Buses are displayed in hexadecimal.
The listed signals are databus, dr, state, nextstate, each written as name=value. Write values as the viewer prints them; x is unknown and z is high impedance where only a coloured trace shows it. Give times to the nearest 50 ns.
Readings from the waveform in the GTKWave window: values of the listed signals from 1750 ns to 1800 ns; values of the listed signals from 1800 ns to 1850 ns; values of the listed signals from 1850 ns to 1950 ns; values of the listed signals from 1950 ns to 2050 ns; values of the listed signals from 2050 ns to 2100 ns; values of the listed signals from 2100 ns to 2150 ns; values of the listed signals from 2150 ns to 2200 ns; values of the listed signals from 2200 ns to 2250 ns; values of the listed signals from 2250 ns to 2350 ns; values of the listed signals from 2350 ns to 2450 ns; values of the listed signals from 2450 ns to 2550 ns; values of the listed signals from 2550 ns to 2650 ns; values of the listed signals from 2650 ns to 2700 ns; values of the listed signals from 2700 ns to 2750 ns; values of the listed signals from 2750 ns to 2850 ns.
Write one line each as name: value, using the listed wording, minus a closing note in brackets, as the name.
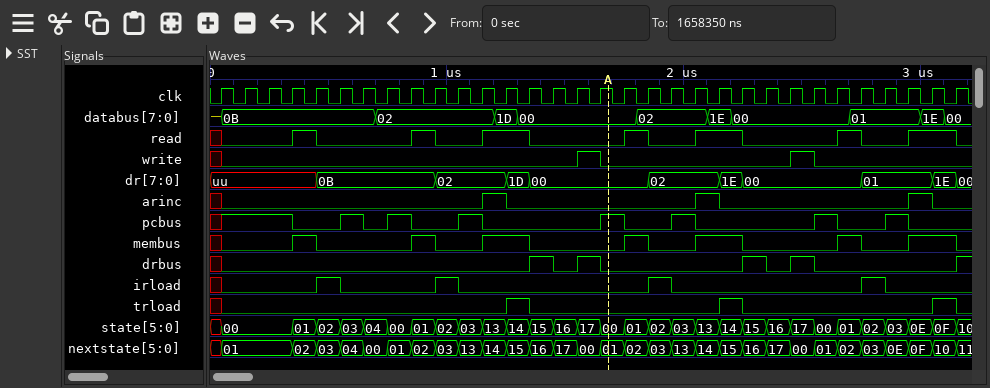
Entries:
values of the listed signals from 1750 ns to 1800 ns: databus=00, dr=00, state=01, nextstate=02
values of the listed signals from 1800 ns to 1850 ns: databus=02, dr=00, state=01, nextstate=02
values of the listed signals from 1850 ns to 1950 ns: databus=02, dr=02, state=02, nextstate=03
values of the listed signals from 1950 ns to 2050 ns: databus=02, dr=02, state=03, nextstate=13
values of the listed signals from 2050 ns to 2100 ns: databus=02, dr=02, state=13, nextstate=14
values of the listed signals from 2100 ns to 2150 ns: databus=1E, dr=02, state=13, nextstate=14
values of the listed signals from 2150 ns to 2200 ns: databus=1E, dr=1E, state=14, nextstate=15
values of the listed signals from 2200 ns to 2250 ns: databus=00, dr=1E, state=14, nextstate=15
values of the listed signals from 2250 ns to 2350 ns: databus=00, dr=00, state=15, nextstate=16
values of the listed signals from 2350 ns to 2450 ns: databus=00, dr=00, state=16, nextstate=17
values of the listed signals from 2450 ns to 2550 ns: databus=00, dr=00, state=17, nextstate=00
values of the listed signals from 2550 ns to 2650 ns: databus=00, dr=00, state=00, nextstate=01
values of the listed signals from 2650 ns to 2700 ns: databus=00, dr=00, state=01, nextstate=02
values of the listed signals from 2700 ns to 2750 ns: databus=01, dr=00, state=01, nextstate=02
values of the listed signals from 2750 ns to 2850 ns: databus=01, dr=01, state=02, nextstate=03
